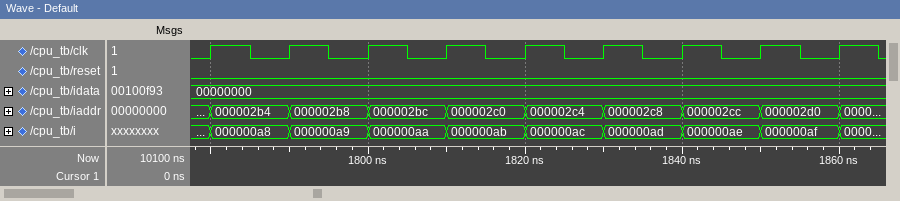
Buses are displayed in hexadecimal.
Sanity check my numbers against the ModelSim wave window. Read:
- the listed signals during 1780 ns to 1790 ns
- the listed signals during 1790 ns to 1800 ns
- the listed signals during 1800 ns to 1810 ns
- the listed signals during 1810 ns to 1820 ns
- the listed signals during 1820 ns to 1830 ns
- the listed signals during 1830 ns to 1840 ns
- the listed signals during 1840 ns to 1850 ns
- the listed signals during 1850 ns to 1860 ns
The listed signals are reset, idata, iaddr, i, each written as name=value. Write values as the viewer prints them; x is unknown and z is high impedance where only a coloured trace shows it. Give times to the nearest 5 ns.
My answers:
reset=0, idata=00000000, iaddr=000002b4, i=000000a8
reset=0, idata=00000000, iaddr=000002b8, i=000000a9
reset=0, idata=00000000, iaddr=000002bc, i=000000aa
reset=0, idata=00000000, iaddr=000002c0, i=000000ab
reset=0, idata=00000000, iaddr=000002c4, i=000000ac
reset=0, idata=00000000, iaddr=000002c8, i=000000ad
reset=0, idata=00000000, iaddr=000002cc, i=000000ae
reset=0, idata=00000000, iaddr=000002d0, i=000000af
